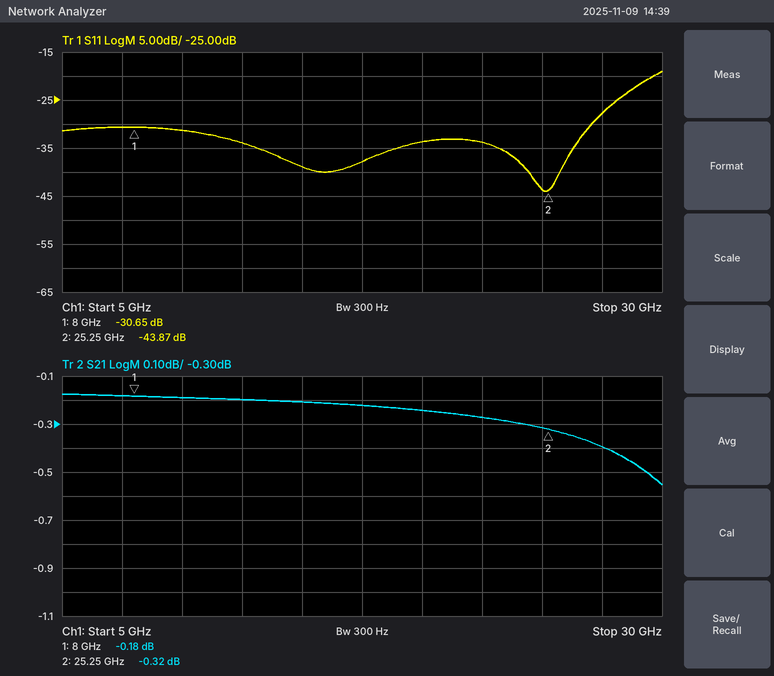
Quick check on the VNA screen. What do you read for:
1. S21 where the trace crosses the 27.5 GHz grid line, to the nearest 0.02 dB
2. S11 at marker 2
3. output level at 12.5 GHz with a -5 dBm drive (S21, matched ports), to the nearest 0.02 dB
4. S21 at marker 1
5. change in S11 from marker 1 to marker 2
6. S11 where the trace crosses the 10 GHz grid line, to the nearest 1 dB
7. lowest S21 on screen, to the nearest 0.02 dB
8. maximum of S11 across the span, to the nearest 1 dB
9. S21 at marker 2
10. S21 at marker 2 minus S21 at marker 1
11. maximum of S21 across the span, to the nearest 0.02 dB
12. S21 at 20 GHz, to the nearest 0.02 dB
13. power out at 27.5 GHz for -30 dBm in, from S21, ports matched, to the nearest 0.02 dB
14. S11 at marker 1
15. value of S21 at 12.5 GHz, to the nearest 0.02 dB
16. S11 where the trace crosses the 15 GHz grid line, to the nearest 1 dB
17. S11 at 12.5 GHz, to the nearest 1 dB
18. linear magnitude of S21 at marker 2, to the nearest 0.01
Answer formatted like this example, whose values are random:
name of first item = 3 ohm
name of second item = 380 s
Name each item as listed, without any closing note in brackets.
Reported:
S21 where the trace crosses the 27.5 GHz grid line, to the nearest 0.02 dB = -0.40 dB
S11 at marker 2 = -43.87 dB
output level at 12.5 GHz with a -5 dBm drive (S21, matched ports), to the nearest 0.02 dB = -5.20 dBm
S21 at marker 1 = -0.18 dB
change in S11 from marker 1 to marker 2 = -13.22 dB
S11 where the trace crosses the 10 GHz grid line, to the nearest 1 dB = -31 dB
lowest S21 on screen, to the nearest 0.02 dB = -0.56 dB
maximum of S11 across the span, to the nearest 1 dB = -19 dB
S21 at marker 2 = -0.32 dB
S21 at marker 2 minus S21 at marker 1 = -0.14 dB
maximum of S21 across the span, to the nearest 0.02 dB = -0.18 dB
S21 at 20 GHz, to the nearest 0.02 dB = -0.24 dB
power out at 27.5 GHz for -30 dBm in, from S21, ports matched, to the nearest 0.02 dB = -30.40 dBm
S11 at marker 1 = -30.65 dB
value of S21 at 12.5 GHz, to the nearest 0.02 dB = -0.20 dB
S11 where the trace crosses the 15 GHz grid line, to the nearest 1 dB = -39 dB
S11 at 12.5 GHz, to the nearest 1 dB = -34 dB
linear magnitude of S21 at marker 2, to the nearest 0.01 = 0.96
